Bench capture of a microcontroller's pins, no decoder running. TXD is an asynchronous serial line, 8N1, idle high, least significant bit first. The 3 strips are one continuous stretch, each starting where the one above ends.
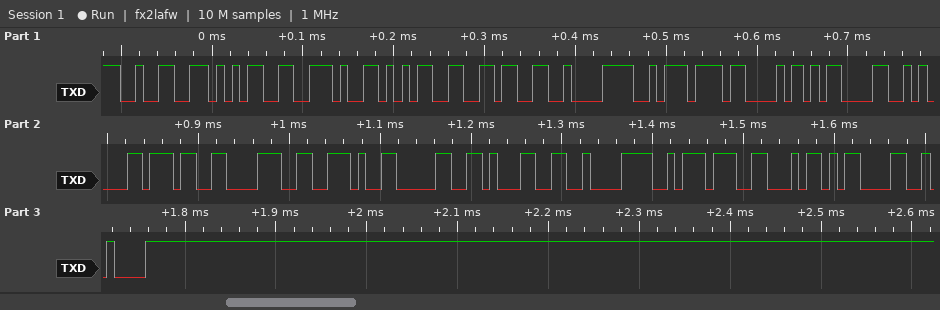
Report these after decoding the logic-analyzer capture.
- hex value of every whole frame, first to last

0x32 0x35 0x2E 0x35 0x36 0xC2 0xBA 0x43 0x0D 0x0A 0x37 0x38 0x2E 0x30 0x31 0xC2 0xBA 0x46 0x0D 0x0A
